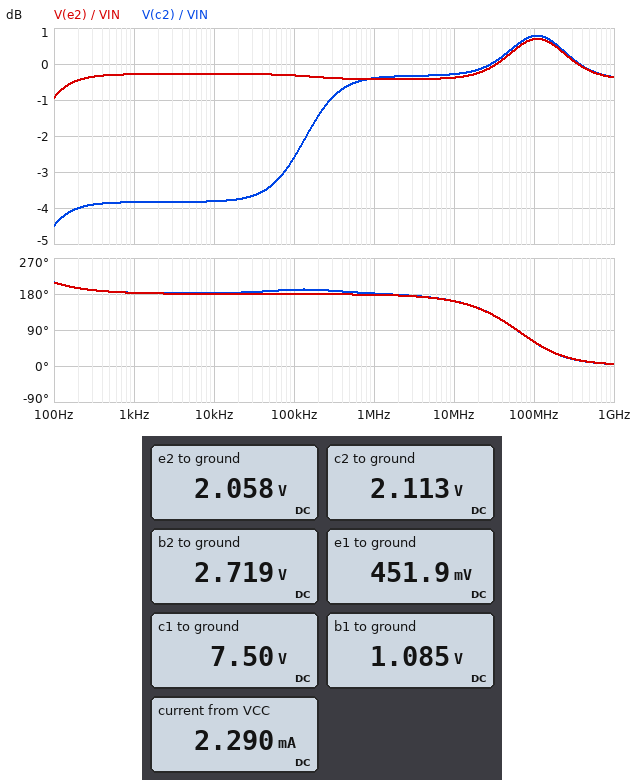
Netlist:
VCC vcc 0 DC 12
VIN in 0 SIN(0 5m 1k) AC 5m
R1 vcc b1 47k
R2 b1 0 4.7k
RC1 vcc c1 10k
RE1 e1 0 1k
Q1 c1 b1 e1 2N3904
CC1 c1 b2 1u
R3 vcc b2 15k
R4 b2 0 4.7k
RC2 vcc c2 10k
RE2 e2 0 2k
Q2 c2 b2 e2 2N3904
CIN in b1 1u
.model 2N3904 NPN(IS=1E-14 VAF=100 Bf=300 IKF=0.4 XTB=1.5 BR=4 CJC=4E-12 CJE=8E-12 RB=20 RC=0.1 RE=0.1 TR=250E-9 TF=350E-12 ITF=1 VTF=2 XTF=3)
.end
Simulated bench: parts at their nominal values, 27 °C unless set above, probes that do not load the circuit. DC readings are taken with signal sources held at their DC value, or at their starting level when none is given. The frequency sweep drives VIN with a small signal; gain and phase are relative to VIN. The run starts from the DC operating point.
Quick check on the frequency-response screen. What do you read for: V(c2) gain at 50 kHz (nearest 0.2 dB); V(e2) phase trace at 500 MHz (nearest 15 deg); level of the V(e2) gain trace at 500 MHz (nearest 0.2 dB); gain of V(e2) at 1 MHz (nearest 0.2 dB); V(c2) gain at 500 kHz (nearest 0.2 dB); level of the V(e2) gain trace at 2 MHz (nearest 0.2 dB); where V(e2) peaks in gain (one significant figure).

-3.4 dB
15 deg
-0.2 dB
-0.4 dB
-0.6 dB
-0.4 dB
100 MHz
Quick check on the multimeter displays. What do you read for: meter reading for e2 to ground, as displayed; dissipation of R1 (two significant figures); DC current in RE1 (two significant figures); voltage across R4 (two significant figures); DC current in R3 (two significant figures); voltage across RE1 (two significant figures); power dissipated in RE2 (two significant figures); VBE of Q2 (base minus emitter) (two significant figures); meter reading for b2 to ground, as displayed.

2.058 V
2.5 mW
450 µA
2.7 V
620 µA
450 mV
2.1 mW
660 mV
2.719 V
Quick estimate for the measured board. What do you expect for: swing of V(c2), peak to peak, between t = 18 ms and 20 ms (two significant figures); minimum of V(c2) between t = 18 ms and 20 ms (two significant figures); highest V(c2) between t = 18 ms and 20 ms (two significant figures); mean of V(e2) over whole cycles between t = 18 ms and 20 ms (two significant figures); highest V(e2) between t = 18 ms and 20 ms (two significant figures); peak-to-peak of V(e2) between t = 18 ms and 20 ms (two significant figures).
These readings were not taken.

6.4 mV
2.1 V
2.1 V
2.1 V
2.1 V
9.7 mV
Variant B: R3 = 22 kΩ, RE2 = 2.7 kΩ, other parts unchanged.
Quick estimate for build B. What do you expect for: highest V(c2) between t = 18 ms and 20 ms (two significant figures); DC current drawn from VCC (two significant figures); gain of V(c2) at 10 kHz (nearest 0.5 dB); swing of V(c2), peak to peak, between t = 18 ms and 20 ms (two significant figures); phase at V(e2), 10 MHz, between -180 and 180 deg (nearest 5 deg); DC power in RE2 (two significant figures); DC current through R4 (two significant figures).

6.6 V
1.7 mA
19.5 dB
95 mV
140 deg
800 µW
450 µA
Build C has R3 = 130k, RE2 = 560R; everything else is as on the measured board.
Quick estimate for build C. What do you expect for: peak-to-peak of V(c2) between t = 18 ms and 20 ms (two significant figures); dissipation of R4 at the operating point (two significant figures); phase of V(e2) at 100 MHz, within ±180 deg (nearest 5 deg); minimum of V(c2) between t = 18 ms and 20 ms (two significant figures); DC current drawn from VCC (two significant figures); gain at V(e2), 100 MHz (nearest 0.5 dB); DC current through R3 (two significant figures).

1.4 mV
37 µW
85 deg
12 V
770 µA
-4.0 dB
89 µA
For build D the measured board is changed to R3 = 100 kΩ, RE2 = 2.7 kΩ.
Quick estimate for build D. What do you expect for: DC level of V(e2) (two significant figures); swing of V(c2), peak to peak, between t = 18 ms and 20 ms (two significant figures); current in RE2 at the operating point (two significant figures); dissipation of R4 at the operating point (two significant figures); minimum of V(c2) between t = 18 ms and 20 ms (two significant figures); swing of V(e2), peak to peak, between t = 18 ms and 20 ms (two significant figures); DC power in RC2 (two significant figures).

17 mV
43 mV
6.4 µA
62 µW
12 V
12 mV
400 nW
